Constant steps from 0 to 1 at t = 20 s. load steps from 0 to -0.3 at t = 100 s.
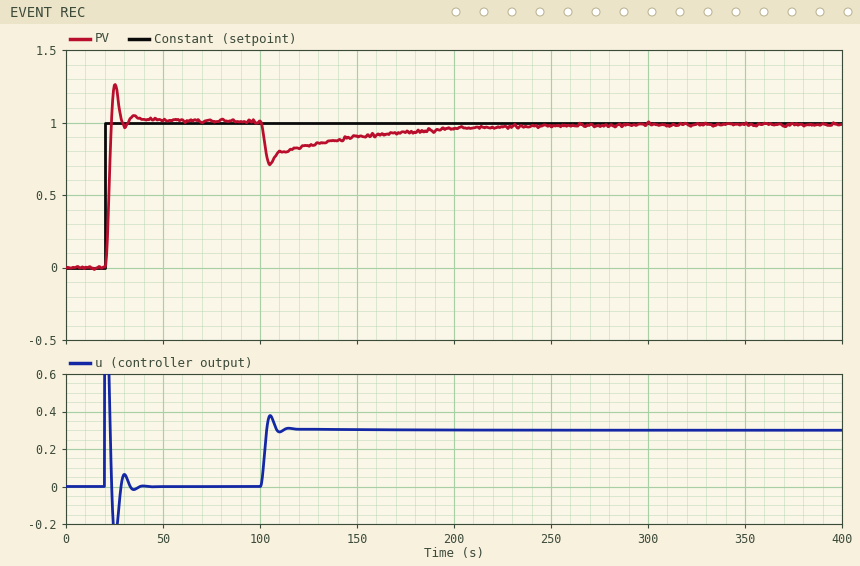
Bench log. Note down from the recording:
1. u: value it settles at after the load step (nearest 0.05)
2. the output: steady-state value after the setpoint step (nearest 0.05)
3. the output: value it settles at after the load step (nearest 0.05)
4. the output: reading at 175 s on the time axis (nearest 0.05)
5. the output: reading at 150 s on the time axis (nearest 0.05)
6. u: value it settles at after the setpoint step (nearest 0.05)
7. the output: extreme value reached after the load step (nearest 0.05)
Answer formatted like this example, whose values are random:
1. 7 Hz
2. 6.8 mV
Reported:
1. 0.30
2. 1.00
3. 1.00
4. 0.95
5. 0.90
6. 0.00
7. 0.70
